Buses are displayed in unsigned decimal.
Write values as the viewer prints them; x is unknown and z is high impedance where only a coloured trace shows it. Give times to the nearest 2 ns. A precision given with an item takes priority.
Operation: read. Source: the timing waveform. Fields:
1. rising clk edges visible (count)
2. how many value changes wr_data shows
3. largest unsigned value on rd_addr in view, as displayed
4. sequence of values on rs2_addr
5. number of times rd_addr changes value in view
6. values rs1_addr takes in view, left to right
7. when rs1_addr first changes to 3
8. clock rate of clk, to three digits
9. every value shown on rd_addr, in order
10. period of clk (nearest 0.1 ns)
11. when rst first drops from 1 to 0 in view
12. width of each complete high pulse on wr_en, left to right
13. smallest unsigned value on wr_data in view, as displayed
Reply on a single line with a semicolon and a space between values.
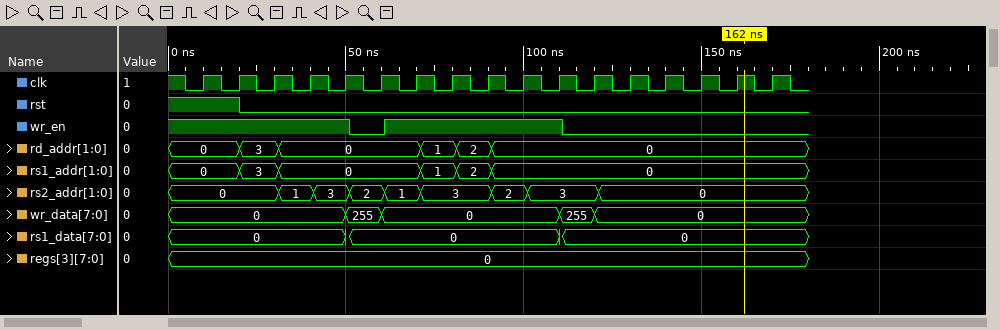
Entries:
17; 4; 3; 0, 1, 3, 2, 1, 3, 2, 3, 0; 5; 0, 3, 0, 1, 2, 0; 20 ns; 100 MHz; 0, 3, 0, 1, 2, 0; 10 ns; 20 ns; 50 ns; 0
